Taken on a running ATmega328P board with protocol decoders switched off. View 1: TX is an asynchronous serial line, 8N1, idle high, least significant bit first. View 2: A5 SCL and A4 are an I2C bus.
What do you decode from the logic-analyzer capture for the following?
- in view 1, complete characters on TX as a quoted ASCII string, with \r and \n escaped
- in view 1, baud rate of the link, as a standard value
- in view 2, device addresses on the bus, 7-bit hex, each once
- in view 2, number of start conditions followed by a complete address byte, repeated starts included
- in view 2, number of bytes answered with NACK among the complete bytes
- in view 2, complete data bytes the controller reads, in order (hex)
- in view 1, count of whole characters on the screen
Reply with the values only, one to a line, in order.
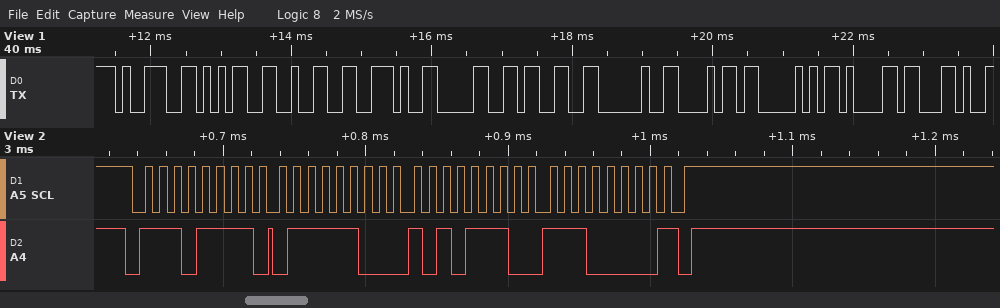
"952.03 hPa,"
9600 baud
0x77
1
1
7C AE E0
11
